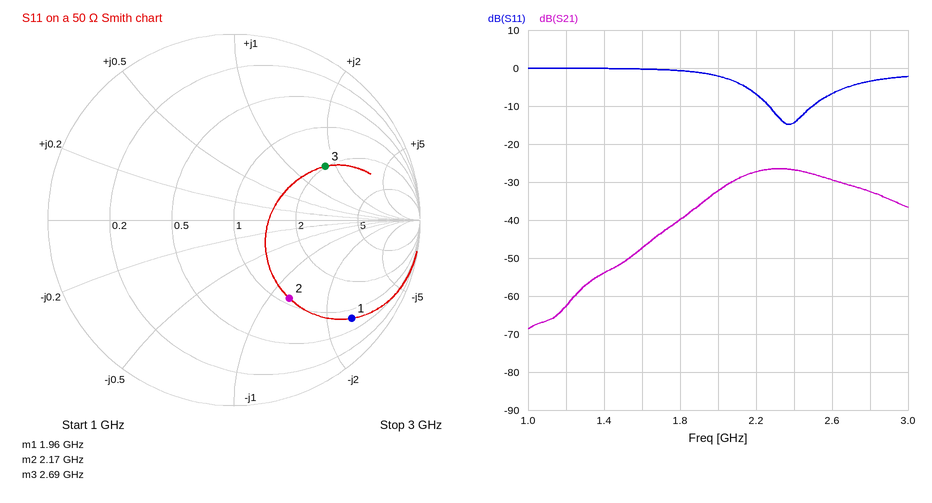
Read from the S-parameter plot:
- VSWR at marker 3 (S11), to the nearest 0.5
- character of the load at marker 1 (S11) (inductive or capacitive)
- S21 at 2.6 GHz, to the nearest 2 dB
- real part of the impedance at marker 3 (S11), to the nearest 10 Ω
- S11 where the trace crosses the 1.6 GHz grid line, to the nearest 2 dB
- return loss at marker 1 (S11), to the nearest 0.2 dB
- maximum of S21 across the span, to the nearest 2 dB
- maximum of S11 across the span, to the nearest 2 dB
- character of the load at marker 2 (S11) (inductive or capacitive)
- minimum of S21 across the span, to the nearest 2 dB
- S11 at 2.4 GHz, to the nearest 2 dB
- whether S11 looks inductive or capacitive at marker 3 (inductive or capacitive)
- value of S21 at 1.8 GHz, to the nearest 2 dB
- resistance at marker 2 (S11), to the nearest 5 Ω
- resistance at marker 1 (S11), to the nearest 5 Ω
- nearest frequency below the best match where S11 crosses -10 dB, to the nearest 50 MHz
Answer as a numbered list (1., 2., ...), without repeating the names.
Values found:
1. 3.5
2. capacitive
3. -30 dB
4. 100 Ω
5. 0 dB
6. 1.6 dB
7. -26 dB
8. 0 dB
9. capacitive
10. -68 dB
11. -14 dB
12. inductive
13. -40 dB
14. 55 Ω
15. 40 Ω
16. 2.25 GHz
